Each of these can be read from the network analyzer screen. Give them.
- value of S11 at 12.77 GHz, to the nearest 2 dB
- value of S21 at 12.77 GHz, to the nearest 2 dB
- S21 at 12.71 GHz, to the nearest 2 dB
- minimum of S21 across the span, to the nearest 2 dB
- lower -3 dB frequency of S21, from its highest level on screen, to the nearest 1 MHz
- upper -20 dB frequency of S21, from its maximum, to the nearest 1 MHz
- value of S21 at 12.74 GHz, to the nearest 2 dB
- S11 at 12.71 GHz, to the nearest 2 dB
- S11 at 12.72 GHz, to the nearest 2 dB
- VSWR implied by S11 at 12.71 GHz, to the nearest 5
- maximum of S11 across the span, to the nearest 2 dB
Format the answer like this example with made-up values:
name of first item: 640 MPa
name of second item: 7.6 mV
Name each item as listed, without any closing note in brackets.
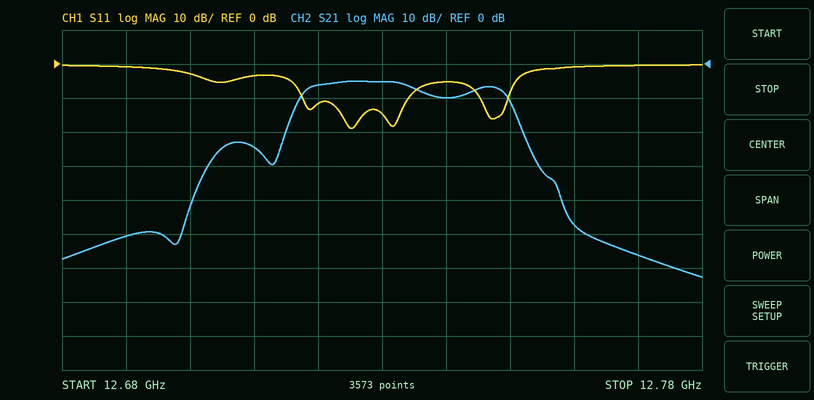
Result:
value of S11 at 12.77 GHz, to the nearest 2 dB: 0 dB
value of S21 at 12.77 GHz, to the nearest 2 dB: -56 dB
S21 at 12.71 GHz, to the nearest 2 dB: -24 dB
minimum of S21 across the span, to the nearest 2 dB: -62 dB
lower -3 dB frequency of S21, from its highest level on screen, to the nearest 1 MHz: 12.718 GHz
upper -20 dB frequency of S21, from its maximum, to the nearest 1 MHz: 12.753 GHz
value of S21 at 12.74 GHz, to the nearest 2 dB: -10 dB
S11 at 12.71 GHz, to the nearest 2 dB: -4 dB
S11 at 12.72 GHz, to the nearest 2 dB: -12 dB
VSWR implied by S11 at 12.71 GHz, to the nearest 5: 5
maximum of S11 across the span, to the nearest 2 dB: 0 dB
